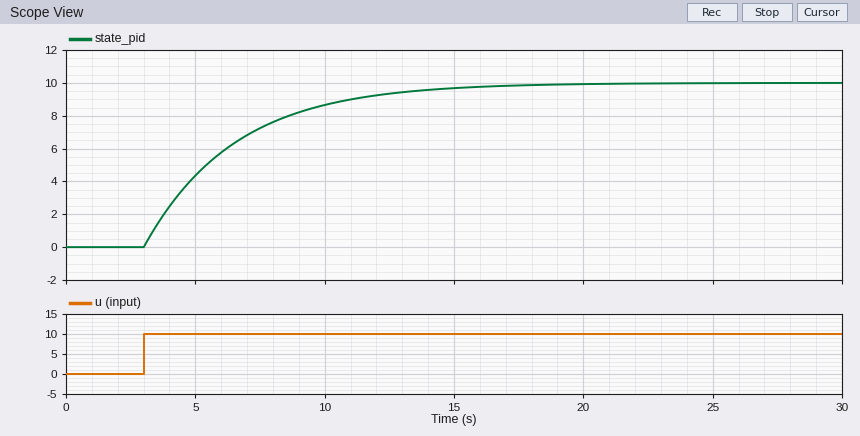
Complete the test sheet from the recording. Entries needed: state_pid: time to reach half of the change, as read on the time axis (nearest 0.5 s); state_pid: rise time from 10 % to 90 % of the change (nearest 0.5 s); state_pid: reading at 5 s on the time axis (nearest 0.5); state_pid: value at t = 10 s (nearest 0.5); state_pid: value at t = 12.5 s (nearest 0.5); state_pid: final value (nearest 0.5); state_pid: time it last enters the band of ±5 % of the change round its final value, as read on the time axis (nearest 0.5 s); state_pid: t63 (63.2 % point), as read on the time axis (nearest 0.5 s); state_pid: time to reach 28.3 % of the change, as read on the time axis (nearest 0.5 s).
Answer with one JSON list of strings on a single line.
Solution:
["5.5 s", "7.5 s", "4.5", "8.5", "9.5", "10.0", "13.5 s", "6.5 s", "4.0 s"]
